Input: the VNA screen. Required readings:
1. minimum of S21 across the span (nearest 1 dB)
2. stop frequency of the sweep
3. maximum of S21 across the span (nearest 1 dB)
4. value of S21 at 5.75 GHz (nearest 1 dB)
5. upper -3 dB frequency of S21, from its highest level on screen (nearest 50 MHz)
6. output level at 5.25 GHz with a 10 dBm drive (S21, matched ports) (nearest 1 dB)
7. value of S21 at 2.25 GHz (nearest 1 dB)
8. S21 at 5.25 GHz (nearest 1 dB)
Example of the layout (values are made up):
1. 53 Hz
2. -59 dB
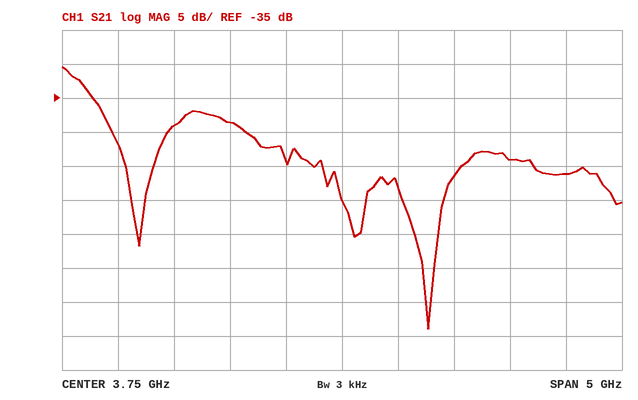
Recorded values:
1. -69 dB
2. 6.25 GHz
3. -30 dB
4. -46 dB
5. 1.45 GHz
6. -34 dBm
7. -39 dB
8. -44 dB
